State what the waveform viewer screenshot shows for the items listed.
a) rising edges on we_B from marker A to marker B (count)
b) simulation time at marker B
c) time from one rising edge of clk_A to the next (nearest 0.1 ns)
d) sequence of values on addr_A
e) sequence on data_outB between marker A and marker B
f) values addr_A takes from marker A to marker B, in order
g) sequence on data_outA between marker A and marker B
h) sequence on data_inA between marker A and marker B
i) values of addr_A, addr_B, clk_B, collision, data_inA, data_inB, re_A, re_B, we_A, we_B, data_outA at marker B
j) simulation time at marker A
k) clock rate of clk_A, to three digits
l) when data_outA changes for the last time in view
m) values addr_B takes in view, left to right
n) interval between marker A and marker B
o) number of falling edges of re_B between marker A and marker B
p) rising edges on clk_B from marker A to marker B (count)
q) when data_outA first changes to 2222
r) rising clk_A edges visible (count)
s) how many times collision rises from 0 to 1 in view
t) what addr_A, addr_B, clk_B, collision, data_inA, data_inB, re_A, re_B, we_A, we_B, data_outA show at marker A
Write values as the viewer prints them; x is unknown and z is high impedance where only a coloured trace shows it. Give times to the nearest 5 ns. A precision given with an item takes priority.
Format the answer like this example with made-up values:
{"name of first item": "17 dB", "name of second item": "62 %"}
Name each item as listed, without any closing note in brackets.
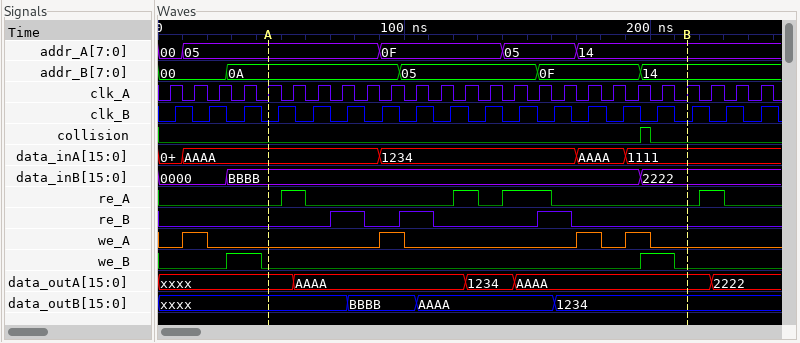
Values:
{"rising edges on we_B from marker A to marker B": "1", "simulation time at marker B": "215 ns", "time from one rising edge of clk_A to the next": "10 ns", "sequence of values on addr_A": "00, 05, 0F, 05, 14", "sequence on data_outB between marker A and marker B": "xxxx, BBBB, AAAA, 1234", "values addr_A takes from marker A to marker B, in order": "05, 0F, 05, 14", "sequence on data_outA between marker A and marker B": "xxxx, AAAA, 1234, AAAA", "sequence on data_inA between marker A and marker B": "AAAA, 1234, AAAA, 1111", "values of addr_A, addr_B, clk_B, collision, data_inA, data_inB, re_A, re_B, we_A, we_B, data_outA at marker B": "addr_A=14, addr_B=14, clk_B=0, collision=0, data_inA=1111, data_inB=2222, re_A=0, re_B=0, we_A=0, we_B=0, data_outA=AAAA", "simulation time at marker A": "45 ns", "clock rate of clk_A, to three digits": "100 MHz", "when data_outA changes for the last time in view": "225 ns", "values addr_B takes in view, left to right": "00, 0A, 05, 0F, 14", "interval between marker A and marker B": "170 ns", "number of falling edges of re_B between marker A and marker B": "3", "rising edges on clk_B from marker A to marker B": "12", "when data_outA first changes to 2222": "225 ns", "rising clk_A edges visible": "25", "how many times collision rises from 0 to 1 in view": "1", "what addr_A, addr_B, clk_B, collision, data_inA, data_inB, re_A, re_B, we_A, we_B, data_outA show at marker A": "addr_A=05, addr_B=0A, clk_B=0, collision=0, data_inA=AAAA, data_inB=BBBB, re_A=0, re_B=0, we_A=0, we_B=0, data_outA=xxxx"}
